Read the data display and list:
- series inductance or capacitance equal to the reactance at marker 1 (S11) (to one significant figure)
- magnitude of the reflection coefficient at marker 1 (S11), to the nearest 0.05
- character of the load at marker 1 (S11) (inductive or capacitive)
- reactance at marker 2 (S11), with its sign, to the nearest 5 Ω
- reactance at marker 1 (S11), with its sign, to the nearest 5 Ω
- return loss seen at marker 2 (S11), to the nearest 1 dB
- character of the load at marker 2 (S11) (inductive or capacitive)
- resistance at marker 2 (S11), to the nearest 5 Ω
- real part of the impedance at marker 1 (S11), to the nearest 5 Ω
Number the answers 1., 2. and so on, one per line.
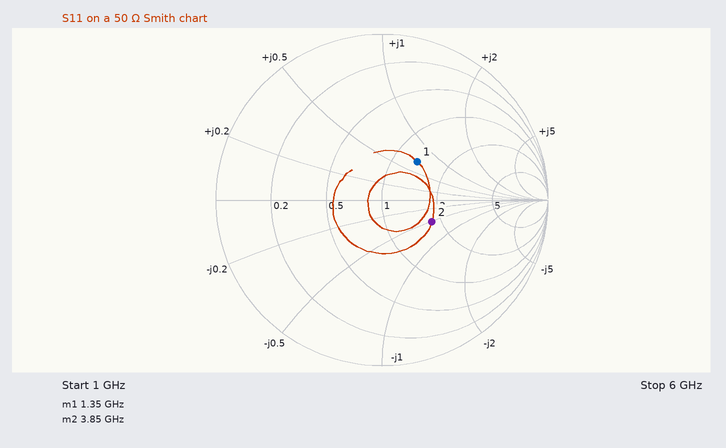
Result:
1. 4 nH
2. 0.30
3. inductive
4. -25 Ω
5. +35 Ω
6. 10 dB
7. capacitive
8. 90 Ω
9. 65 Ω
